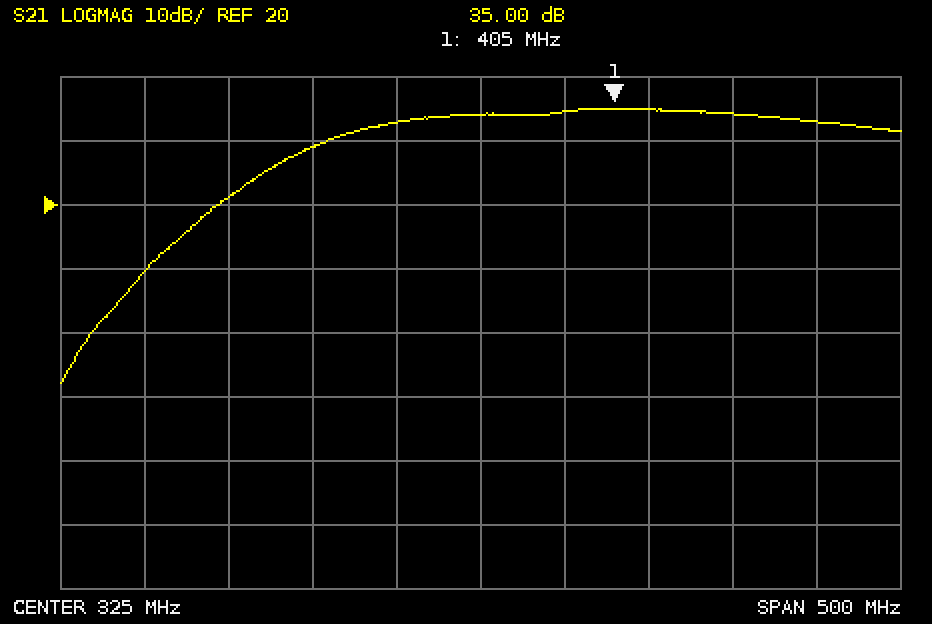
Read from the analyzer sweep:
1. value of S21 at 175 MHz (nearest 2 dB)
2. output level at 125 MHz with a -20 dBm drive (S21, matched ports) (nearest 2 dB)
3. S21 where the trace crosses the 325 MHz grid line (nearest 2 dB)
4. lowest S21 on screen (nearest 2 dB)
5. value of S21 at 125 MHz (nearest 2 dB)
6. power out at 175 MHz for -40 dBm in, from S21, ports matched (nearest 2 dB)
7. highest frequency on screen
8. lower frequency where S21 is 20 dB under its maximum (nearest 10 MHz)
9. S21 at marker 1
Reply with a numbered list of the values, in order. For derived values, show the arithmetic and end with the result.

1. 22 dB
2. -20 dBm + (10 dB) = -10 dBm
3. 34 dB
4. -8 dB
5. 10 dB
6. -40 dBm + (22 dB) = -18 dBm
7. 575 MHz
8. 150 MHz
9. 35.00 dB
